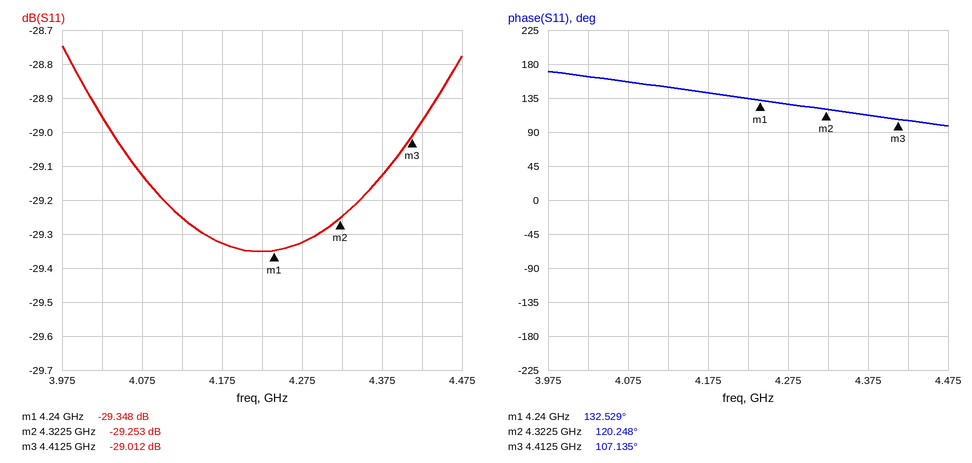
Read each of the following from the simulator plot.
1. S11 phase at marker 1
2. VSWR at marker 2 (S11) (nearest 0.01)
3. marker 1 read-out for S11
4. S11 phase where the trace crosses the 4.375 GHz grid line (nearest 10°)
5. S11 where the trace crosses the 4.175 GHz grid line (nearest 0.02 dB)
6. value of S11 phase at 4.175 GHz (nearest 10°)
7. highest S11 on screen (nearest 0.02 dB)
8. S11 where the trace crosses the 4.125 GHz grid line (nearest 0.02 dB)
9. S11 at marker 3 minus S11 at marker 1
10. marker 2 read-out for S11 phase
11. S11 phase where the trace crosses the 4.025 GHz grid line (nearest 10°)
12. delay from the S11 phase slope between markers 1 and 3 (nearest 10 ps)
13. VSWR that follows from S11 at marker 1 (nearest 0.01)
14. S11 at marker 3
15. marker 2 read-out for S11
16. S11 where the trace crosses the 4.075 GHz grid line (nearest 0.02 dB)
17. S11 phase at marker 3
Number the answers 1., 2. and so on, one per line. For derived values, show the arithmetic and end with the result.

1. 132.529°
2. (1 + 0.0345)/(1 − 0.0345) ≈ 1.07
3. -29.348 dB
4. 110°
5. -29.32 dB
6. 140°
7. -28.74 dB
8. -29.26 dB
9. -29.012 − (-29.348) = 0.336 dB
10. 120.248°
11. 160°
12. −(107.135° − (132.529°))/(360° × 172.5 MHz) ≈ 409 ps, so 410 ps to the nearest 10 ps
13. (1 + 0.0341)/(1 − 0.0341) ≈ 1.07
14. -29.012 dB
15. -29.253 dB
16. -29.12 dB
17. 107.135°
